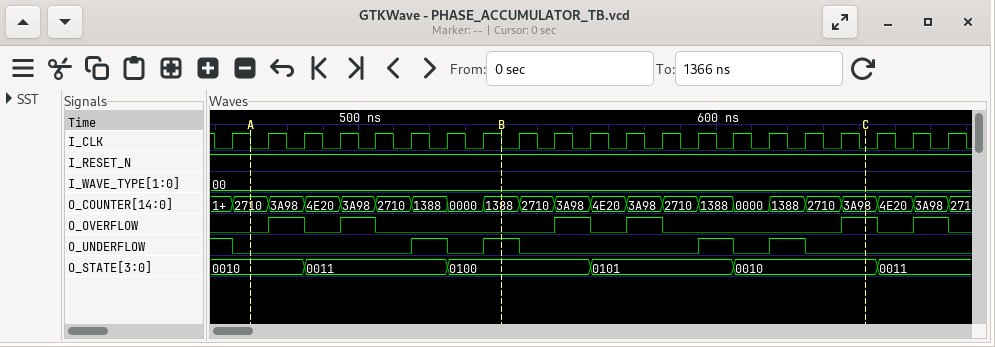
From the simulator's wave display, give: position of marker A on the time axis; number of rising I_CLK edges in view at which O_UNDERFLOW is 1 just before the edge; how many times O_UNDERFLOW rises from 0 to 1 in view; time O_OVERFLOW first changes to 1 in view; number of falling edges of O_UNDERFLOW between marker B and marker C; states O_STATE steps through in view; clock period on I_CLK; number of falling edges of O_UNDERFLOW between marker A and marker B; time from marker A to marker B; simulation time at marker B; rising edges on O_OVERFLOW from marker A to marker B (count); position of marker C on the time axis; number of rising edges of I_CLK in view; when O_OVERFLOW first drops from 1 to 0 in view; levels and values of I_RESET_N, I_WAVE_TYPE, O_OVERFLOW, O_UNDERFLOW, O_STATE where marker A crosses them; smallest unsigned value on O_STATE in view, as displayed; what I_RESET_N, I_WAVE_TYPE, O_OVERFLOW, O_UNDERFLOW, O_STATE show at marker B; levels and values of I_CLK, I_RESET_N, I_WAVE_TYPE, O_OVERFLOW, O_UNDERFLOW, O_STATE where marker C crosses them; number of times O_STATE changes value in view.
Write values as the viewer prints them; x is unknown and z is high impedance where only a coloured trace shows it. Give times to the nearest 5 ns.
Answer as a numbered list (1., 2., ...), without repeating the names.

1. 470 ns
2. 5
3. 4
4. 475 ns
5. 3
6. 0010, 0011, 0100, 0101, 0010, 0011
7. 10 ns
8. 1
9. 70 ns
10. 540 ns
11. 2
12. 640 ns
13. 21
14. 485 ns
15. I_RESET_N=1, I_WAVE_TYPE=00, O_OVERFLOW=0, O_UNDERFLOW=0, O_STATE=0010
16. 0010
17. I_RESET_N=1, I_WAVE_TYPE=00, O_OVERFLOW=0, O_UNDERFLOW=1, O_STATE=0100
18. I_CLK=0, I_RESET_N=1, I_WAVE_TYPE=00, O_OVERFLOW=1, O_UNDERFLOW=0, O_STATE=0010
19. 5
